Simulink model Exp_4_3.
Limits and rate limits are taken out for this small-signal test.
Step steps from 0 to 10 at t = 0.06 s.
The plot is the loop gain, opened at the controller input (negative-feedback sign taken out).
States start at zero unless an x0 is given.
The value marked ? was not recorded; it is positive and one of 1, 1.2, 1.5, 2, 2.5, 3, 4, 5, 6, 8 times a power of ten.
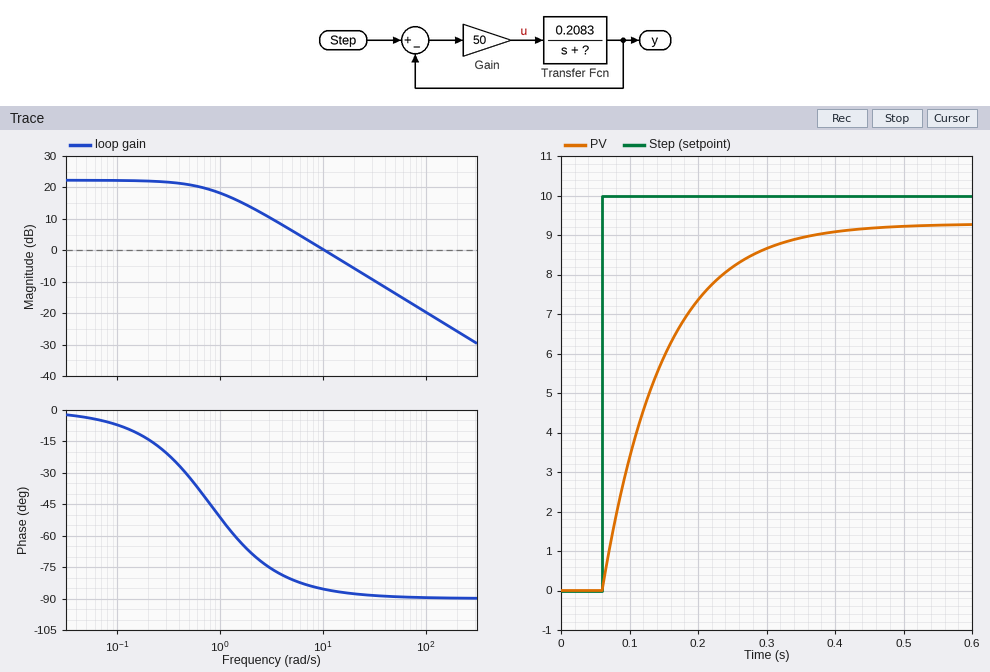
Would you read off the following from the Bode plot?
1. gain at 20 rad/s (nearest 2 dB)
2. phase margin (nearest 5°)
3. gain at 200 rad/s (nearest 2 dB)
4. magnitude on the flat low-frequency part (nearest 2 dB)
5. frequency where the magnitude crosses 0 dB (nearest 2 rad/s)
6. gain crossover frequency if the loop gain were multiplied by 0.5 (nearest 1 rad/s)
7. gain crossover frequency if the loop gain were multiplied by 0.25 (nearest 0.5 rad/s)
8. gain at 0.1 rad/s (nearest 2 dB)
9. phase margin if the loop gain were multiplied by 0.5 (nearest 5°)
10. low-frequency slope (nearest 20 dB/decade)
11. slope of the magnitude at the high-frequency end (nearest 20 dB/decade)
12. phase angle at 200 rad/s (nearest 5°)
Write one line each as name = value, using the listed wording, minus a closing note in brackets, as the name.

gain at 20 rad/s = -6 dB
phase margin = 95°
gain at 200 rad/s = -26 dB
magnitude on the flat low-frequency part = 22 dB
frequency where the magnitude crosses 0 dB = 10 rad/s
gain crossover frequency if the loop gain were multiplied by 0.5 = 5 rad/s
gain crossover frequency if the loop gain were multiplied by 0.25 = 2.5 rad/s
gain at 0.1 rad/s = 22 dB
phase margin if the loop gain were multiplied by 0.5 = 100°
low-frequency slope = 0 dB/decade
slope of the magnitude at the high-frequency end = -20 dB/decade
phase angle at 200 rad/s = -90°
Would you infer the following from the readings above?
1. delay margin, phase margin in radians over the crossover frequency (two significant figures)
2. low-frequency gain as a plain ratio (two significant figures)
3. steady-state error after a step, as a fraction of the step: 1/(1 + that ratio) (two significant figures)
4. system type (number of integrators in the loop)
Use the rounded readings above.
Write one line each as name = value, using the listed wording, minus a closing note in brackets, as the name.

delay margin, phase margin in radians over the crossover frequency = 0.17 s
low-frequency gain as a plain ratio = 13
steady-state error after a step, as a fraction of the step: 1/(1 + that ratio) = 0.071
system type = 0
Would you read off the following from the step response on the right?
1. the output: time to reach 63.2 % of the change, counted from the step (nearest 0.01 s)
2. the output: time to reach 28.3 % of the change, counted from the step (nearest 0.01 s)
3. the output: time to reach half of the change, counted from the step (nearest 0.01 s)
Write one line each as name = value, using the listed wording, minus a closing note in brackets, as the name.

the output: time to reach 63.2 % of the change, counted from the step = 0.09 s
the output: time to reach 28.3 % of the change, counted from the step = 0.03 s
the output: time to reach half of the change, counted from the step = 0.06 s
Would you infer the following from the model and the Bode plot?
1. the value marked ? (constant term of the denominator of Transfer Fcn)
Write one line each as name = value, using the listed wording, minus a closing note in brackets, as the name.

the value marked ? = 0.8
